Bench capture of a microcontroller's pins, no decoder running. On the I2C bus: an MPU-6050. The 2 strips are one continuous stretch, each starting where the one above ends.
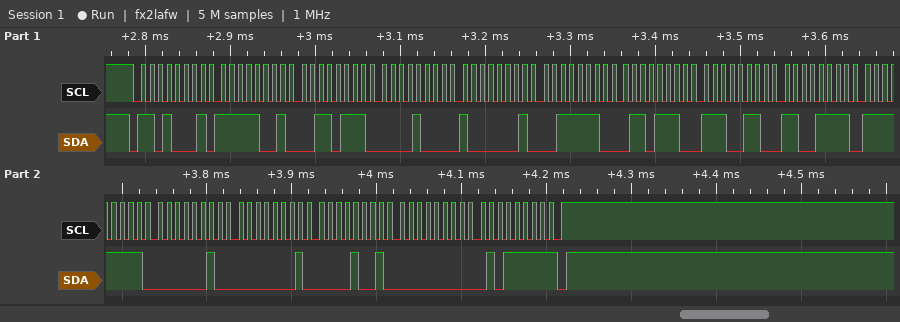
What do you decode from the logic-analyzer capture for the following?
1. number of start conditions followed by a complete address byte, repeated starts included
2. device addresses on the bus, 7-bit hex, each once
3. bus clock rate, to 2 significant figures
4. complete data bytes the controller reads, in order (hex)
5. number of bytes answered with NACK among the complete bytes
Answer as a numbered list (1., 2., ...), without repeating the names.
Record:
1. 1
2. 0x68
3. 100 kHz
4. F9 37 08 81 3E 6E E6 CF FF 02 01 09 00 5F
5. 1
